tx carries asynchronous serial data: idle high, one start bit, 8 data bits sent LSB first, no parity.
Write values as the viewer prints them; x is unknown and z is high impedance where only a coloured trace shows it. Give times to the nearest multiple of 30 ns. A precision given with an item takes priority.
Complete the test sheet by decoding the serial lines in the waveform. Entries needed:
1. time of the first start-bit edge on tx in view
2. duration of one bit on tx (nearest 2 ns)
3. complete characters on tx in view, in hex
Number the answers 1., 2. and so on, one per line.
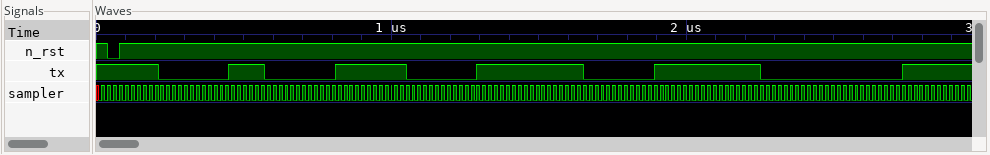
1. 210 ns
2. 120 ns
3. 32, 0E
